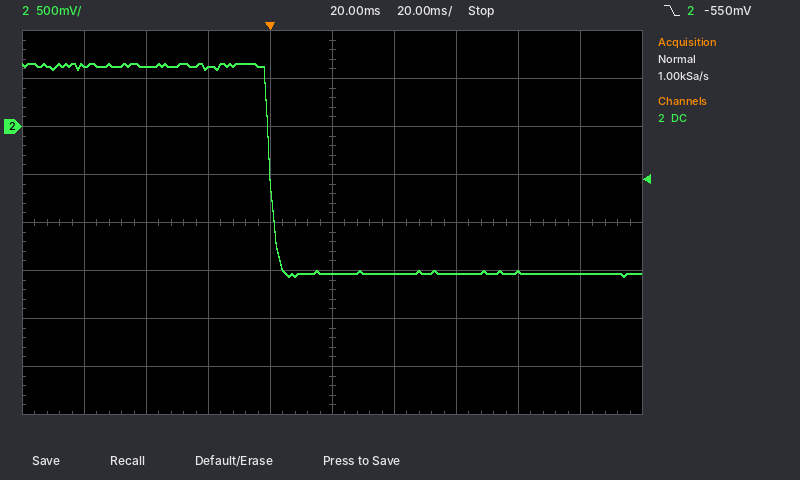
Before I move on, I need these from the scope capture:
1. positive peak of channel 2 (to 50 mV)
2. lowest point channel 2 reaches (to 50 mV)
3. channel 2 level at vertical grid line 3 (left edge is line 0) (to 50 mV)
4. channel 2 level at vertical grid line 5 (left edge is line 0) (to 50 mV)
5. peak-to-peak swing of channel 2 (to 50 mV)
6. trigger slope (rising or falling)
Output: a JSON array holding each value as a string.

["650 mV", "-1.55 V", "600 mV", "-1.55 V", "2.20 V", "falling"]
